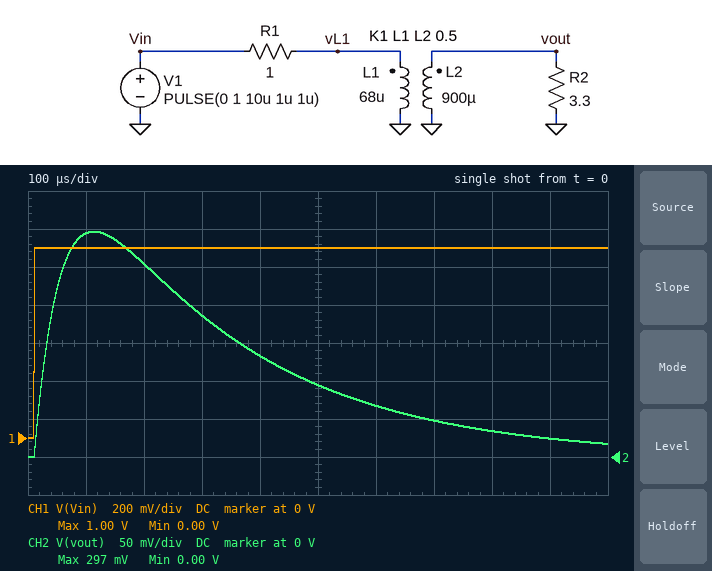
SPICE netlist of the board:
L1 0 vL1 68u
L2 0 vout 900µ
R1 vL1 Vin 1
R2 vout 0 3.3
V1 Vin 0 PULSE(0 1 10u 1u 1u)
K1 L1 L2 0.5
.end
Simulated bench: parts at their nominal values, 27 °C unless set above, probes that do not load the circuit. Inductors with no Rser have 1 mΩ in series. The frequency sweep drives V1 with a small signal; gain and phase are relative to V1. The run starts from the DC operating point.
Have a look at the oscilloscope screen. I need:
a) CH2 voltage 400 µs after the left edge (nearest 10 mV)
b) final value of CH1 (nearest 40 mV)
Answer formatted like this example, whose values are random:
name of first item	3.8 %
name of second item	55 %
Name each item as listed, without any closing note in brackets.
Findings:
CH2 voltage 400 µs after the left edge	130 mV
final value of CH1	1.00 V
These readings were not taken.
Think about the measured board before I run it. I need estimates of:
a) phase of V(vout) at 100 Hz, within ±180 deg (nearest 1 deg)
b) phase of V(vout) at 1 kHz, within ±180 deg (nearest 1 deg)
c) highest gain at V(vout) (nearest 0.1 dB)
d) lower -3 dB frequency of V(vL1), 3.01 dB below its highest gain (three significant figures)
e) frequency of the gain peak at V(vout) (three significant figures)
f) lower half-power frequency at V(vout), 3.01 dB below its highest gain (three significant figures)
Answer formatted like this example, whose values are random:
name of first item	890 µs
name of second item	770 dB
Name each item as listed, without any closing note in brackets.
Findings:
phase of V(vout) at 100 Hz, within ±180 deg	78 deg
phase of V(vout) at 1 kHz, within ±180 deg	12 deg
highest gain at V(vout)	-8.8 dB
lower -3 dB frequency of V(vL1), 3.01 dB below its highest gain	3.27 kHz
frequency of the gain peak at V(vout)	1.35 kHz
lower half-power frequency at V(vout), 3.01 dB below its highest gain	422 Hz
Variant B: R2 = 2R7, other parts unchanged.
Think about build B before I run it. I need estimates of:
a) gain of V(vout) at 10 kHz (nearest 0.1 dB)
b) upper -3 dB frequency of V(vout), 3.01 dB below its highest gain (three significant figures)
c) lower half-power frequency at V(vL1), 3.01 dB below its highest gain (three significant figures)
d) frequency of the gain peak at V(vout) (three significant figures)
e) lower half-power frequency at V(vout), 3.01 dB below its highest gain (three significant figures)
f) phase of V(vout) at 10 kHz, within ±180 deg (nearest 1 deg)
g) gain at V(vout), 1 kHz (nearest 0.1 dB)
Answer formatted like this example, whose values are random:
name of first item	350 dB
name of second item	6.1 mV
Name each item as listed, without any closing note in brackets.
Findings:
gain of V(vout) at 10 kHz	-19.2 dB
upper -3 dB frequency of V(vout), 3.01 dB below its highest gain	4.12 kHz
lower half-power frequency at V(vL1), 3.01 dB below its highest gain	3.25 kHz
frequency of the gain peak at V(vout)	1.22 kHz
lower half-power frequency at V(vout), 3.01 dB below its highest gain	362 Hz
phase of V(vout) at 10 kHz, within ±180 deg	-69 deg
gain at V(vout), 1 kHz	-10.3 dB
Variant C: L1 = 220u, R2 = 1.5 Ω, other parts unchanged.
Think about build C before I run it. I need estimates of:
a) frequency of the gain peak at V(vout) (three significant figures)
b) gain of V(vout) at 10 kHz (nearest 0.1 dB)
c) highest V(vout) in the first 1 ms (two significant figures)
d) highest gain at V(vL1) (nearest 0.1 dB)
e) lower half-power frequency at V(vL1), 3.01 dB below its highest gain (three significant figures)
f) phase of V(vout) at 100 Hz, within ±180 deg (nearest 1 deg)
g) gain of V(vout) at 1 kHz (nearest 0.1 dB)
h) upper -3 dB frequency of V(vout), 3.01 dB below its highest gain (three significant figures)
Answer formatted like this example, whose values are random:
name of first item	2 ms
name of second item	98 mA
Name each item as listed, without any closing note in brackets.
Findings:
frequency of the gain peak at V(vout)	506 Hz
gain of V(vout) at 10 kHz	-29.0 dB
highest V(vout) in the first 1 ms	220 mV
highest gain at V(vL1)	0 dB
lower half-power frequency at V(vL1), 3.01 dB below its highest gain	1.02 kHz
phase of V(vout) at 100 Hz, within ±180 deg	62 deg
gain of V(vout) at 1 kHz	-12.5 dB
upper -3 dB frequency of V(vout), 3.01 dB below its highest gain	1.49 kHz
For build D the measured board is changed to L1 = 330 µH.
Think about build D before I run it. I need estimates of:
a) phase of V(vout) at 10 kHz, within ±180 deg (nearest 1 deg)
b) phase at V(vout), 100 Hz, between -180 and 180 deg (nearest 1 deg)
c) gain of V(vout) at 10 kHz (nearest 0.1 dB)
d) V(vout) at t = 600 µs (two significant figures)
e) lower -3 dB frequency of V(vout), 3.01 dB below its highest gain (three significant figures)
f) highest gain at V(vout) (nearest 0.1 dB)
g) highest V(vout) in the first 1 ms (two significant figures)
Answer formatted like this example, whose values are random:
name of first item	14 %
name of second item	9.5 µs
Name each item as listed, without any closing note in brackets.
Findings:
phase of V(vout) at 10 kHz, within ±180 deg	-82 deg
phase at V(vout), 100 Hz, between -180 and 180 deg	69 deg
gain of V(vout) at 10 kHz	-23.9 dB
V(vout) at t = 600 µs	230 mV
lower -3 dB frequency of V(vout), 3.01 dB below its highest gain	228 Hz
highest gain at V(vout)	-6.9 dB
highest V(vout) in the first 1 ms	350 mV
